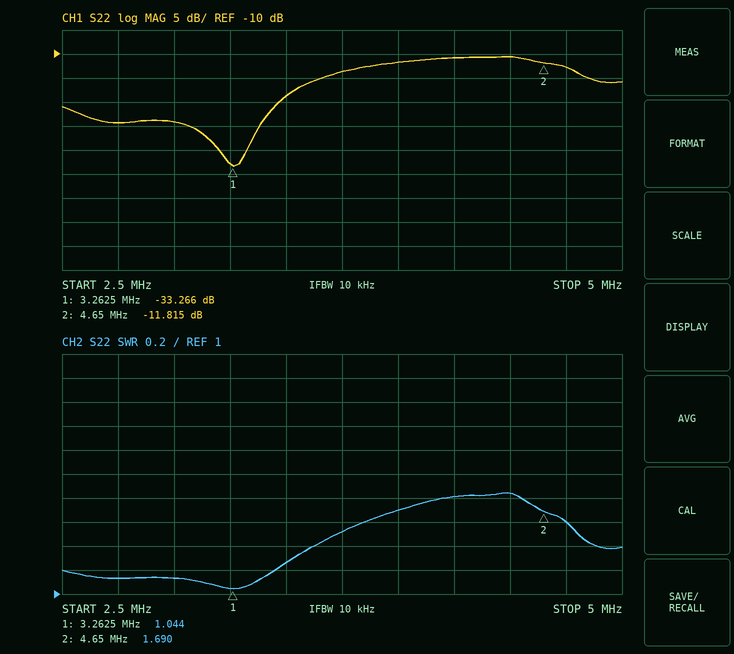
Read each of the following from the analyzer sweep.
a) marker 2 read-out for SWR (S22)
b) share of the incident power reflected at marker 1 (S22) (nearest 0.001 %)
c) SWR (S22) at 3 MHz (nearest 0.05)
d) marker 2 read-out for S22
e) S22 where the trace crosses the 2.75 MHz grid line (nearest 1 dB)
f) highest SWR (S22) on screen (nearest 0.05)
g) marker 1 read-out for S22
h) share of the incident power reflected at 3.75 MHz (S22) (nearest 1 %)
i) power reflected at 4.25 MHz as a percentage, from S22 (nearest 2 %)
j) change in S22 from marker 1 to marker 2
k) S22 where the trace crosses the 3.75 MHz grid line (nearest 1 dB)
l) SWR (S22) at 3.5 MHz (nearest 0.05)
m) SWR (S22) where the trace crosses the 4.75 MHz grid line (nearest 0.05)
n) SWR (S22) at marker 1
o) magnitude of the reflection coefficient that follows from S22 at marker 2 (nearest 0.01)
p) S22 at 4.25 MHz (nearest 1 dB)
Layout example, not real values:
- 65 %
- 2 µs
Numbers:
- 1.690
- 0.047 %
- 1.15
- -11.815 dB
- -24 dB
- 1.85
- -33.266 dB
- 4 %
- 8 %
- 21.451 dB
- -14 dB
- 1.25
- 1.60
- 1.044
- 0.26
- -11 dB
